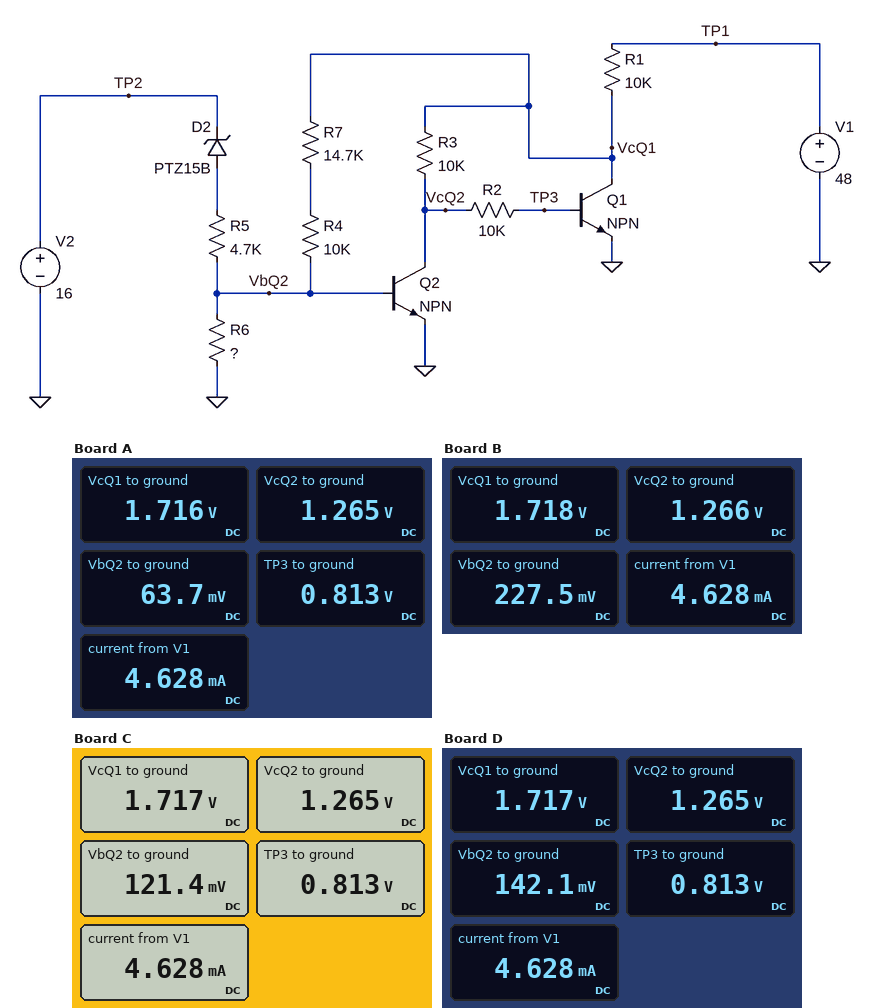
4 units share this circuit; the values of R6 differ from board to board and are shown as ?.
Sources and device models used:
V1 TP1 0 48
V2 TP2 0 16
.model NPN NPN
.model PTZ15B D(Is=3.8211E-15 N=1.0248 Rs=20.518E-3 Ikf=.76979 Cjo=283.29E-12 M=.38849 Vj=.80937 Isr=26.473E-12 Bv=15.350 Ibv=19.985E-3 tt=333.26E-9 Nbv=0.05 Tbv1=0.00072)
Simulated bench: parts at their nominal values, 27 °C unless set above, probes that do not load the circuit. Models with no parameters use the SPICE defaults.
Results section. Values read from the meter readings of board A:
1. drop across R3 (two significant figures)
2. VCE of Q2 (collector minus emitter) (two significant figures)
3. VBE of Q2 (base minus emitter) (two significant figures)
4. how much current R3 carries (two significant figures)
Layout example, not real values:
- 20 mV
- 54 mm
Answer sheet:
- 450 mV
- 1.3 V
- 64 mV
- 45 µA
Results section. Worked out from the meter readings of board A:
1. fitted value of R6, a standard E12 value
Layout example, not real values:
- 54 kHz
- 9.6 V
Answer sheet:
- 330 Ω
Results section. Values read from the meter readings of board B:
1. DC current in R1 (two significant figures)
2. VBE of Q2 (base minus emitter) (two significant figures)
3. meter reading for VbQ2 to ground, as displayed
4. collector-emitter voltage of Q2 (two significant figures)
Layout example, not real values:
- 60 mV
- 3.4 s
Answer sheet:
- 4.6 mA
- 230 mV
- 227.5 mV
- 1.3 V
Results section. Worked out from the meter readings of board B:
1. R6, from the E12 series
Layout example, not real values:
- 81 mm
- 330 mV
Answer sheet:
- 1.5 kΩ
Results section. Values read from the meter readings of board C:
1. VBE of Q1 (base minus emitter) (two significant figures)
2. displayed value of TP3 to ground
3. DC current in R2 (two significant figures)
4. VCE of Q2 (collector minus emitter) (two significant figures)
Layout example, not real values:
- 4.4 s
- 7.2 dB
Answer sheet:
- 810 mV
- 0.813 V
- 45 µA
- 1.3 V
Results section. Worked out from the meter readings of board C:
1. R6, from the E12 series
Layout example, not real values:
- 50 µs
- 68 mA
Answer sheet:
- 680 Ω
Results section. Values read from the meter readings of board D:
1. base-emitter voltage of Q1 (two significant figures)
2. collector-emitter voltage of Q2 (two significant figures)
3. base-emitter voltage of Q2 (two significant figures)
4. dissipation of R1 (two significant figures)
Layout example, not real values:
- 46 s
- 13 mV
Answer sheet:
- 810 mV
- 1.3 V
- 140 mV
- 210 mW
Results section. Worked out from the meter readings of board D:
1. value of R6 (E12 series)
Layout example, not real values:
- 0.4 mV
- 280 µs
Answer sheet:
- 820 Ω
